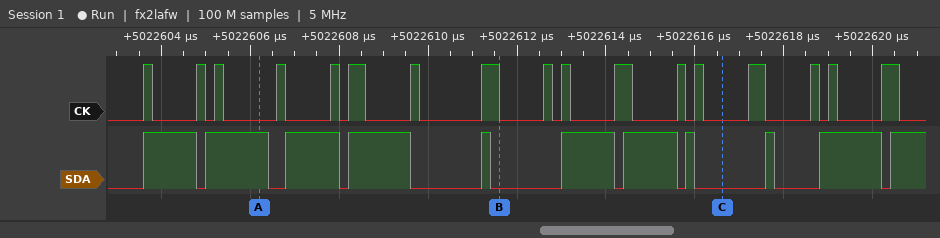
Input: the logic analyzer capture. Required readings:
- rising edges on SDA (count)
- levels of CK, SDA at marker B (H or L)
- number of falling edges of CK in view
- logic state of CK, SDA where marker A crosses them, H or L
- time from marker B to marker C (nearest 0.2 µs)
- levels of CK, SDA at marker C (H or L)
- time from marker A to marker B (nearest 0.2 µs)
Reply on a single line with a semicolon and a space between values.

11; CK=L, SDA=L; 17; CK=L, SDA=H; 5 µs; CK=L, SDA=L; 5.4 µs
